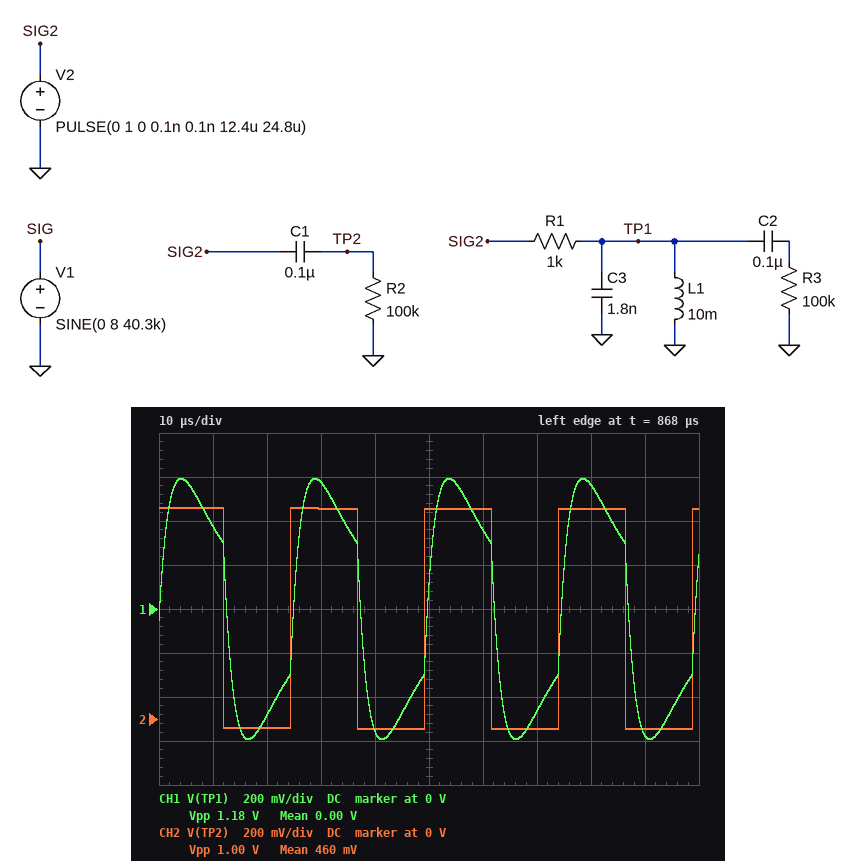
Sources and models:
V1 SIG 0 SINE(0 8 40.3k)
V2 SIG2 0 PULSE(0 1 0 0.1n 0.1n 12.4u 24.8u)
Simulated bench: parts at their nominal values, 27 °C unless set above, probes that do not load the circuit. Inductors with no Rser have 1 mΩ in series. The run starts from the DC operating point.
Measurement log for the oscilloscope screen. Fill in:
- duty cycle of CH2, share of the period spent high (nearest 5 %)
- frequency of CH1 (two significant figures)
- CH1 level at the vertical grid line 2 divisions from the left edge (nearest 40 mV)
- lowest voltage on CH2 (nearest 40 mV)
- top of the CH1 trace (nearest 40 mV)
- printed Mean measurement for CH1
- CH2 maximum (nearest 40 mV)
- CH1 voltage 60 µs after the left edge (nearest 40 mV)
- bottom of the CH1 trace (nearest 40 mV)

50 %
40 kHz
-480 mV
-40 mV
600 mV
0.00 V
960 mV
360 mV
-600 mV
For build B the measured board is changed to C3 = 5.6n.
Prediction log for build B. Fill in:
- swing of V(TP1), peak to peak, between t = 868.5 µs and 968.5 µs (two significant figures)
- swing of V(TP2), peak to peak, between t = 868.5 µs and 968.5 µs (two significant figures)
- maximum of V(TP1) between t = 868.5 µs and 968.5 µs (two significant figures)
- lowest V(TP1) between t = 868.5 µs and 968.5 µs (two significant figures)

850 mV
1.0 V
420 mV
-420 mV
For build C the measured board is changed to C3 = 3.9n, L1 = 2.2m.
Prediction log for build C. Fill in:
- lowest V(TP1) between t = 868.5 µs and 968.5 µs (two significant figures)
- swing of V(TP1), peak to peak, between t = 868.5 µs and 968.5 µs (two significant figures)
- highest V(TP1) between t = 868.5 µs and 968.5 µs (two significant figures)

-570 mV
1.1 V
570 mV
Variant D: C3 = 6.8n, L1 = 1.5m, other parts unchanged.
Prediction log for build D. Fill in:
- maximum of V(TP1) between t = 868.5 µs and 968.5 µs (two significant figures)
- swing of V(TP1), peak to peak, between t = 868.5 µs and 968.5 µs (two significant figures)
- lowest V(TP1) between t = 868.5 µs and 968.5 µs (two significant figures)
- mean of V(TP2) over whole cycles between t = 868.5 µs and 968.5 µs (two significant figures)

510 mV
1.0 V
-510 mV
460 mV
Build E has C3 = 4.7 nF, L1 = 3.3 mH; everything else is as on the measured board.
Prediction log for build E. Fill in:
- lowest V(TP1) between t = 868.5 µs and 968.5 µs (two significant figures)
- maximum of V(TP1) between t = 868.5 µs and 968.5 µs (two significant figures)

-630 mV
630 mV
